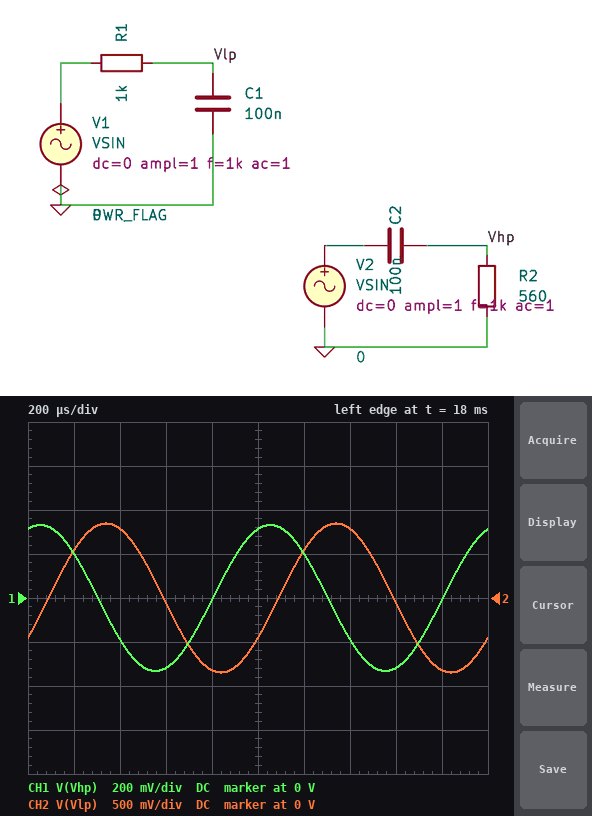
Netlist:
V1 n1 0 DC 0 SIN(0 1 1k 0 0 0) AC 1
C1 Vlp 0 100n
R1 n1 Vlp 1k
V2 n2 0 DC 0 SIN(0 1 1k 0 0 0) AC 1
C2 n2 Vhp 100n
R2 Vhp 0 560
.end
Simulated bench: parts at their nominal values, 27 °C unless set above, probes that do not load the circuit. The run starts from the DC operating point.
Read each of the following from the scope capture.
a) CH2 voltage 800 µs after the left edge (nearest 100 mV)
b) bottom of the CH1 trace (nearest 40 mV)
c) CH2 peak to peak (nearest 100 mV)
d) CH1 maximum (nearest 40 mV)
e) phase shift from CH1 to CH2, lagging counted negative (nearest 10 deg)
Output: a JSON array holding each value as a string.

["-800 mV", "-320 mV", "1.7 V", "320 mV", "-100 deg"]
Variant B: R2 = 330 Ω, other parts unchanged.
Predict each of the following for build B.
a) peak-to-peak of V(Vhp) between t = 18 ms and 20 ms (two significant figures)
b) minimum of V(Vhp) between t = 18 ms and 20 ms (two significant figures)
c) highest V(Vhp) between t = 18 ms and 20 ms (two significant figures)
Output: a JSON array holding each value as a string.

["410 mV", "-200 mV", "200 mV"]
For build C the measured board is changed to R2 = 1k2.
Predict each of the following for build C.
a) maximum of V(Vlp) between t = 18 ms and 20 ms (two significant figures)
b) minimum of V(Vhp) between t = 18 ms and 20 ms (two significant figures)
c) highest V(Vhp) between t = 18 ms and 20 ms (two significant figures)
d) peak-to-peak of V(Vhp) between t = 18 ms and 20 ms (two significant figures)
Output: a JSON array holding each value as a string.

["850 mV", "-600 mV", "600 mV", "1.2 V"]
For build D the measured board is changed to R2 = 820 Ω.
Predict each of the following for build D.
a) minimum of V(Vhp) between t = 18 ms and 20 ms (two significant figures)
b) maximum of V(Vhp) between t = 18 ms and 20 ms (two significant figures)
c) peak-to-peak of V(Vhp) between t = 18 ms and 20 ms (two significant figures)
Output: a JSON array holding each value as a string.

["-460 mV", "460 mV", "920 mV"]
